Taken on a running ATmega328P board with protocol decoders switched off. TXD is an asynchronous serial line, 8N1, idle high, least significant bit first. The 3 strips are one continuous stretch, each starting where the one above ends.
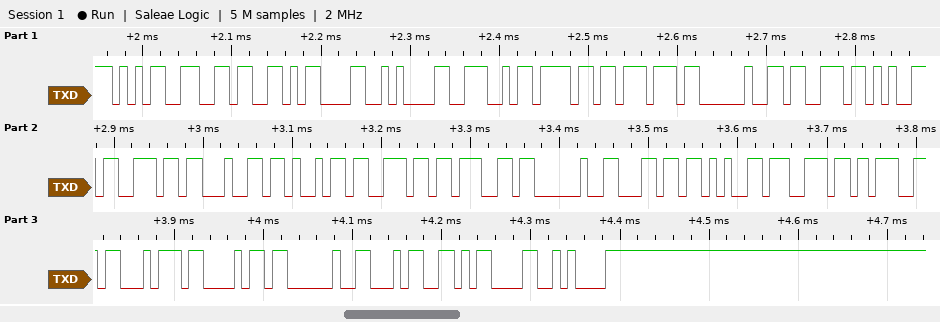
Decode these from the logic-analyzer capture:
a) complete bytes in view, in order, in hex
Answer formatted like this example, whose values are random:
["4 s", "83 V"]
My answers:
["35 36 0D 0A 4E 6F 77 20 73 65 6E 64 69 6E 67 20 6C 65 6E 67 74 68 20 34 0D 0A"]
